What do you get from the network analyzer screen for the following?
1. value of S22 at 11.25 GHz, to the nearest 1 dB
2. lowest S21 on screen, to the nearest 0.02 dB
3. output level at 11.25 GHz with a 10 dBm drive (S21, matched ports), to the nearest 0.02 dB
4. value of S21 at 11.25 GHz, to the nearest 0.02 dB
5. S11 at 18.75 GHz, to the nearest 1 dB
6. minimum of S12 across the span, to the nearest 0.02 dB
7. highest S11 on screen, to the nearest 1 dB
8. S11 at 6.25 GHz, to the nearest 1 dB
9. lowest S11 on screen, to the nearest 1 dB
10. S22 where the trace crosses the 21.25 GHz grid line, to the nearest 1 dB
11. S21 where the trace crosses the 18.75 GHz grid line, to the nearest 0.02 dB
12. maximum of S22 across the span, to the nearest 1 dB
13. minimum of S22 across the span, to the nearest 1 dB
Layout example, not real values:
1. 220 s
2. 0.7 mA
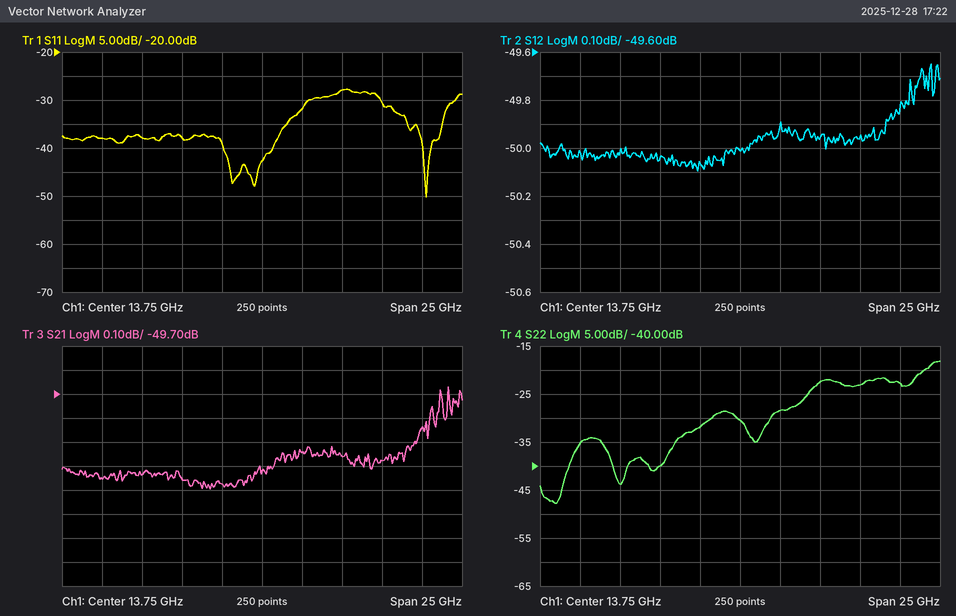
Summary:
1. -32 dB
2. -50.10 dB
3. -40.08 dBm
4. -50.08 dB
5. -28 dB
6. -50.10 dB
7. -28 dB
8. -38 dB
9. -50 dB
10. -23 dB
11. -49.96 dB
12. -18 dB
13. -48 dB
